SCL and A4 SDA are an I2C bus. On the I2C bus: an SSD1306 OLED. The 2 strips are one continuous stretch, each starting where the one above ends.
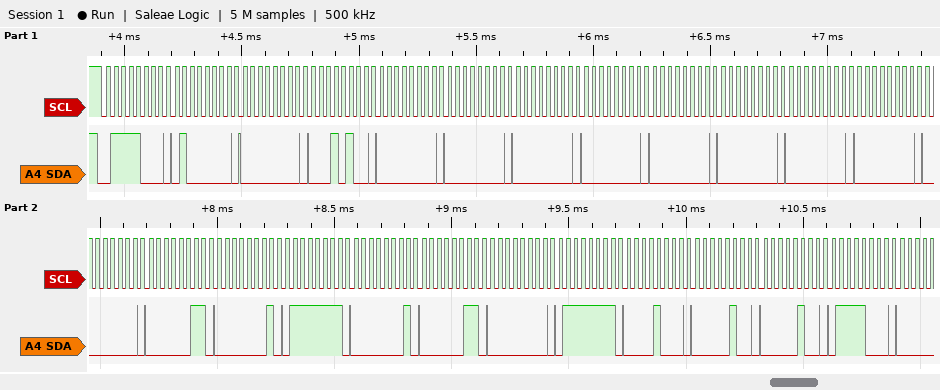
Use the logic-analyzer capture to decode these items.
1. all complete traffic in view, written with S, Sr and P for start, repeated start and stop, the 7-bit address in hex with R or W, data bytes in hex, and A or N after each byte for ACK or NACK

S 3CW A 40 A 00 A 14 A 00 A 00 A 00 A 00 A 00 A 00 A 00 A 00 A 00 A 03 A 01 A 7F A 01 A 03 A 00 A 7F A 08 A 04 A 04 A 78 A
